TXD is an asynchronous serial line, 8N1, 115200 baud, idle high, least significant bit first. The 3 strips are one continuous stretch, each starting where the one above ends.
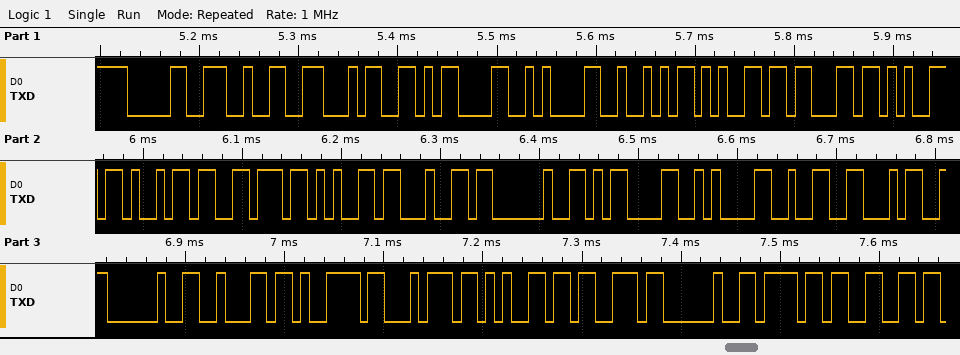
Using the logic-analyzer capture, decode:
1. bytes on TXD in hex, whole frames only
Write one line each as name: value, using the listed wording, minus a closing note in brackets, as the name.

bytes on TXD in hex, whole frames only: 30 32 34 0D 0A 52 65 63 65 69 76 65 64 20 0D 0A 32 34 20 62 79 74 65 73 20 6F 66
